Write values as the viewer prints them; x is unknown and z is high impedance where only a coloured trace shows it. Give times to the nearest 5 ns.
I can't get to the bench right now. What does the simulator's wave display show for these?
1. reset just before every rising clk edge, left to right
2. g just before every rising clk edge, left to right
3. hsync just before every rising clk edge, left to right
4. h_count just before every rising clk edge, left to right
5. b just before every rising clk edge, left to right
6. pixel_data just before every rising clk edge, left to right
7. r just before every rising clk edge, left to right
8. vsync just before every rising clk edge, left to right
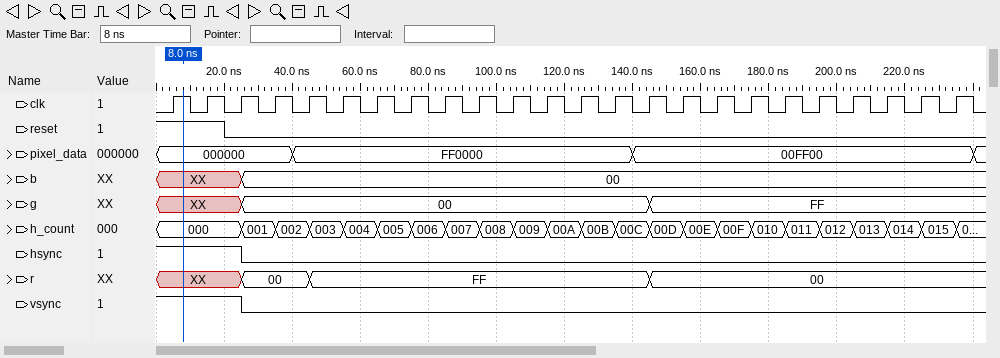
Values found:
1 1 0 0 0 0 0 0 0 0 0 0 0 0 0 0 0 0 0 0 0 0 0 0
XX, XX, XX, 00, 00, 00, 00, 00, 00, 00, 00, 00, 00, 00, 00, FF, FF, FF, FF, FF, FF, FF, FF, FF
1 1 1 0 0 0 0 0 0 0 0 0 0 0 0 0 0 0 0 0 0 0 0 0
000, 000, 000, 001, 002, 003, 004, 005, 006, 007, 008, 009, 00A, 00B, 00C, 00D, 00E, 00F, 010, 011, 012, 013, 014, 015
XX, XX, XX, 00, 00, 00, 00, 00, 00, 00, 00, 00, 00, 00, 00, 00, 00, 00, 00, 00, 00, 00, 00, 00
000000, 000000, 000000, 000000, FF0000, FF0000, FF0000, FF0000, FF0000, FF0000, FF0000, FF0000, FF0000, FF0000, 00FF00, 00FF00, 00FF00, 00FF00, 00FF00, 00FF00, 00FF00, 00FF00, 00FF00, 00FF00
XX, XX, XX, 00, 00, FF, FF, FF, FF, FF, FF, FF, FF, FF, FF, 00, 00, 00, 00, 00, 00, 00, 00, 00
1 1 1 0 0 0 0 0 0 0 0 0 0 0 0 0 0 0 0 0 0 0 0 0
